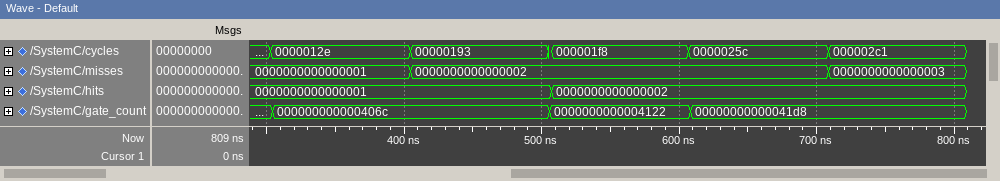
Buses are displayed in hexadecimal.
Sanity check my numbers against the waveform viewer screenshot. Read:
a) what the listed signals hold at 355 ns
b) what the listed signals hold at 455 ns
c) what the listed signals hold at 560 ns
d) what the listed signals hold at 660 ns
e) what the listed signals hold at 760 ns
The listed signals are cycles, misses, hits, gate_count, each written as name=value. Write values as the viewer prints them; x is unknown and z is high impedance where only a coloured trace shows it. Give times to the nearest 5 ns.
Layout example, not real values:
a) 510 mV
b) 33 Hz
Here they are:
a) cycles=0000012e, misses=0000000000000001, hits=0000000000000001, gate_count=000000000000406c
b) cycles=00000193, misses=0000000000000002, hits=0000000000000001, gate_count=000000000000406c
c) cycles=000001f8, misses=0000000000000002, hits=0000000000000002, gate_count=0000000000004122
d) cycles=0000025c, misses=0000000000000002, hits=0000000000000002, gate_count=00000000000041d8
e) cycles=000002c1, misses=0000000000000003, hits=0000000000000002, gate_count=00000000000041d8
